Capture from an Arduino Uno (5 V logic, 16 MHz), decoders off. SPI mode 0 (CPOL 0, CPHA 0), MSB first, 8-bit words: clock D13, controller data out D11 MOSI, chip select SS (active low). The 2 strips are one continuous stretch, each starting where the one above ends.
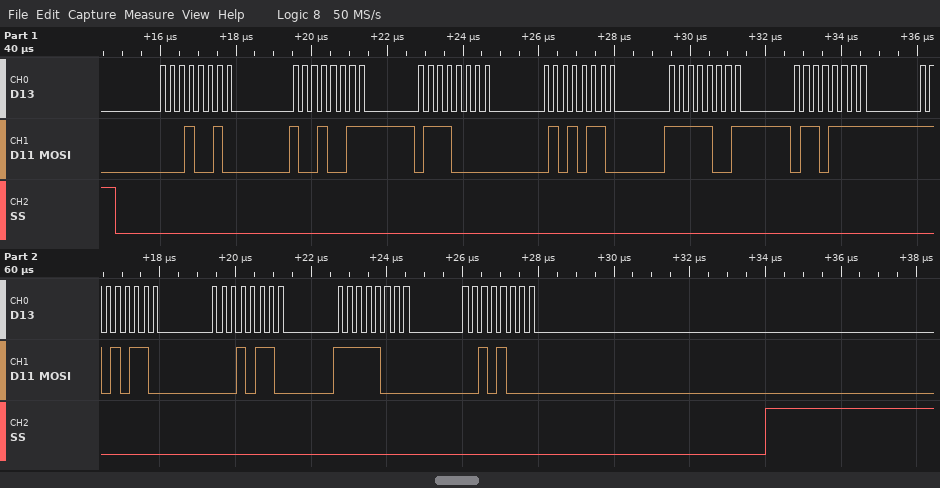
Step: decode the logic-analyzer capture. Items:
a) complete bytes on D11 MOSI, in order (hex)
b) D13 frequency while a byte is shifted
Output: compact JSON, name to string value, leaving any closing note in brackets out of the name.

{"complete bytes on D11 MOSI, in order": "12 93 70 56 F9 6F D6 16 F8 28", "D13 frequency while a byte is shifted": "4 MHz"}
